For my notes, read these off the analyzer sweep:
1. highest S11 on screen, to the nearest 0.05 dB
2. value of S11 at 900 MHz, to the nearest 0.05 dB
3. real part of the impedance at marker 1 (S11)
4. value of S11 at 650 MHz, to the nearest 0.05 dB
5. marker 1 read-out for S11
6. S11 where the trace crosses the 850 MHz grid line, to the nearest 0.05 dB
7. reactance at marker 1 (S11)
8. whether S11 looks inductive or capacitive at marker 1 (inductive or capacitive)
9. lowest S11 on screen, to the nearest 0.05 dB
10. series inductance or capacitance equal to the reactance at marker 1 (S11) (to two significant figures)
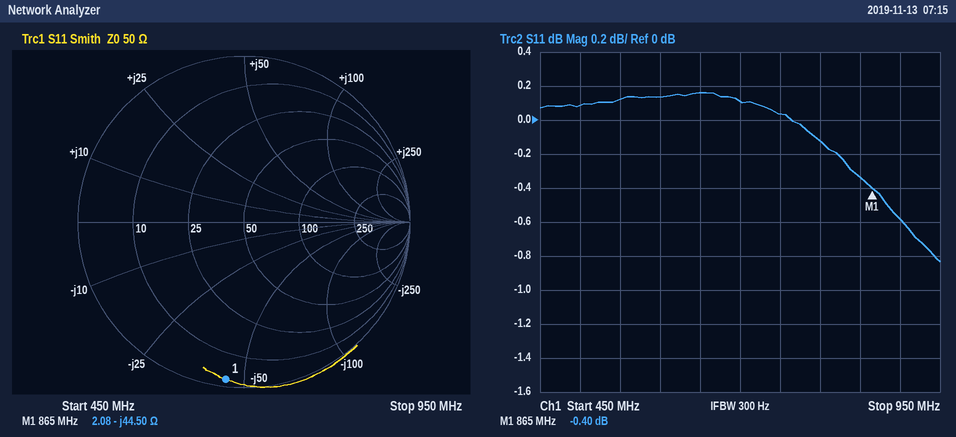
0.15 dB
-0.60 dB
2.08 Ω
0.15 dB
-0.40 dB
-0.35 dB
-44.50 Ω
capacitive
-0.85 dB
4.1 pF
